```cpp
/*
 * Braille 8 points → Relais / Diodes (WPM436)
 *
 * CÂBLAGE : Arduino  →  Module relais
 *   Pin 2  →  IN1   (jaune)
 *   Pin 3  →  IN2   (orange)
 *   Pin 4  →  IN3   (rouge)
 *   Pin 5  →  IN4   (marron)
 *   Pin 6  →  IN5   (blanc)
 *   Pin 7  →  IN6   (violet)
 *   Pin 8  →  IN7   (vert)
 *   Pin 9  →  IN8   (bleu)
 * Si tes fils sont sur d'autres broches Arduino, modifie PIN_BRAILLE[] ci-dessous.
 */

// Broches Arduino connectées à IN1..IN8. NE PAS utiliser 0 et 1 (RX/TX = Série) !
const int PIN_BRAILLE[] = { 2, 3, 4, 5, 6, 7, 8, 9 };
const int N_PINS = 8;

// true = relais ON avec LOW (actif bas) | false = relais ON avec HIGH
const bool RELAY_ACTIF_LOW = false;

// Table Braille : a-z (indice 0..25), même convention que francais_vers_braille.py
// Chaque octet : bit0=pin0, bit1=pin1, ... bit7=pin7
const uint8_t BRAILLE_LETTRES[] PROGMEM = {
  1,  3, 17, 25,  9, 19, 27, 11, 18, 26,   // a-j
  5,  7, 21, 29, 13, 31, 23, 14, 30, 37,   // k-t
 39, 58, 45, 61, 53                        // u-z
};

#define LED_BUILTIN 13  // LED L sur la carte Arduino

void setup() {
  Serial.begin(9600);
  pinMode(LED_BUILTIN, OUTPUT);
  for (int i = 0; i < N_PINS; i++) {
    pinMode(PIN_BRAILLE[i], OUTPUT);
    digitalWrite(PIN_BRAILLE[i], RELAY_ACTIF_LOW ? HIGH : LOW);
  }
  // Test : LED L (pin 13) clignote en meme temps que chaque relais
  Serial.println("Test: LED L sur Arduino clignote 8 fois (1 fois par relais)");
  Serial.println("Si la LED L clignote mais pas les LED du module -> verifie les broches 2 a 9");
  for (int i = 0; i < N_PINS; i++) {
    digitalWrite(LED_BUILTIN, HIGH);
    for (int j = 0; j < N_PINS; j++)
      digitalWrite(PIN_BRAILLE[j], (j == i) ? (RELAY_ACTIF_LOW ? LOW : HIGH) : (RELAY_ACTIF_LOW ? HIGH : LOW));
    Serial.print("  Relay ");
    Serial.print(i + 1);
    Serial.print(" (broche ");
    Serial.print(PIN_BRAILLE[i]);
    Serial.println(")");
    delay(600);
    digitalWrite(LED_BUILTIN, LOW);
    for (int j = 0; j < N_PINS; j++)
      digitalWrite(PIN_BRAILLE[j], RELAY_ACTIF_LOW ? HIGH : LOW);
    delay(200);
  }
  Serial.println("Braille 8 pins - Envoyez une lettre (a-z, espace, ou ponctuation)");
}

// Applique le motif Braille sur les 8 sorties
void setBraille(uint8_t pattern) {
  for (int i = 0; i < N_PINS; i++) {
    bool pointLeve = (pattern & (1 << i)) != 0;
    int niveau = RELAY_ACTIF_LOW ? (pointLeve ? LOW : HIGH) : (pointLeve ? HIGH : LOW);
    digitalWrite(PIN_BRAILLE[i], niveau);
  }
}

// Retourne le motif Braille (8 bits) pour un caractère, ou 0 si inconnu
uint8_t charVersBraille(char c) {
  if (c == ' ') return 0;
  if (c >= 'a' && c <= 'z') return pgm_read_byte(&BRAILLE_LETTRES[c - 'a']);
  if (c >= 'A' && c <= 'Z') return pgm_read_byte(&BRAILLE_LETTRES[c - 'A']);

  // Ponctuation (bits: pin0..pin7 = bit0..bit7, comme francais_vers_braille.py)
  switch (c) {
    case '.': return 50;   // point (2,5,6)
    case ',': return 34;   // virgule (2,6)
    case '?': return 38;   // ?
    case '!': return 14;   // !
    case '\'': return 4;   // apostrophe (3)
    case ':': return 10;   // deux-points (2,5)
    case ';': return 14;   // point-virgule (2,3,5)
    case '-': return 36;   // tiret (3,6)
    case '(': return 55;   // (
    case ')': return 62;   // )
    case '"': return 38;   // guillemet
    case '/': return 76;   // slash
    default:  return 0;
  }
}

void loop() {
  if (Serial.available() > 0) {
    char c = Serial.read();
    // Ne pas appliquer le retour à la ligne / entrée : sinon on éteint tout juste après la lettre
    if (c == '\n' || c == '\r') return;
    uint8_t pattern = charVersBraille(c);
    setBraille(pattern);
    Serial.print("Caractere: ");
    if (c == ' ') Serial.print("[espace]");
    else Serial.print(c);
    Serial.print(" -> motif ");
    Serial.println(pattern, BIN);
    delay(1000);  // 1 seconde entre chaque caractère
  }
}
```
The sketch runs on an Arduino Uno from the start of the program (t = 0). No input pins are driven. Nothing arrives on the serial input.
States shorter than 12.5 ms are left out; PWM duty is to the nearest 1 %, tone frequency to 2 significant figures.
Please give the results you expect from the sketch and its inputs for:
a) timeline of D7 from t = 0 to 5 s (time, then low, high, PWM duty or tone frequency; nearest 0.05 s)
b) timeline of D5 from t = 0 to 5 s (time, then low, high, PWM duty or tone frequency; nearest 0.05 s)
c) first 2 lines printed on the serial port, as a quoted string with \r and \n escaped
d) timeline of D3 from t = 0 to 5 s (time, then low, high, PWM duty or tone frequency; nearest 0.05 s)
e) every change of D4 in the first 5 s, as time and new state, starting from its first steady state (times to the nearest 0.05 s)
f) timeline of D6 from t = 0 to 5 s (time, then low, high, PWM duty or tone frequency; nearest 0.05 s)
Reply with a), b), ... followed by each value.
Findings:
a) 0 s low; 4.1 s high; 4.7 s low
b) 0 s low; 2.5 s high; 3.1 s low
c) "Test: LED L sur Arduino clignote 8 fois (1 fois par relais)\r\nSi la LED L clignote mais pas les LED du module -> verifie les broches 2 a 9\r\n"
d) 0 s low; 0.9 s high; 1.5 s low
e) 0 s low; 1.7 s high; 2.3 s low
f) 0 s low; 3.3 s high; 3.9 s low
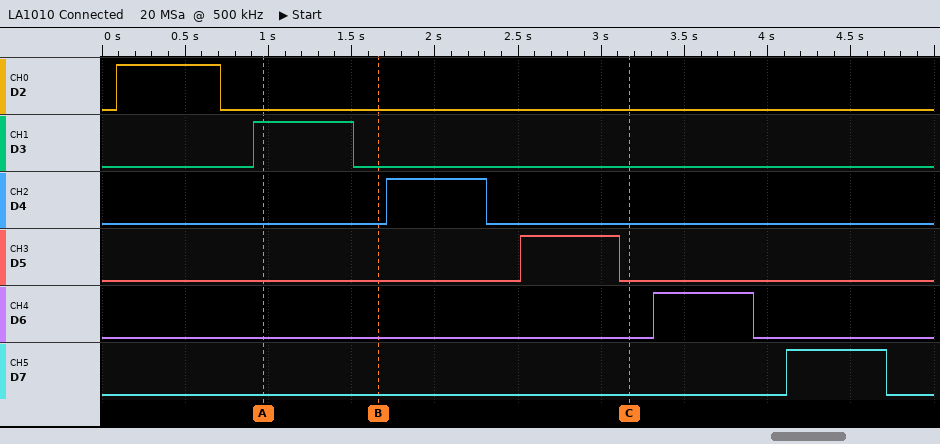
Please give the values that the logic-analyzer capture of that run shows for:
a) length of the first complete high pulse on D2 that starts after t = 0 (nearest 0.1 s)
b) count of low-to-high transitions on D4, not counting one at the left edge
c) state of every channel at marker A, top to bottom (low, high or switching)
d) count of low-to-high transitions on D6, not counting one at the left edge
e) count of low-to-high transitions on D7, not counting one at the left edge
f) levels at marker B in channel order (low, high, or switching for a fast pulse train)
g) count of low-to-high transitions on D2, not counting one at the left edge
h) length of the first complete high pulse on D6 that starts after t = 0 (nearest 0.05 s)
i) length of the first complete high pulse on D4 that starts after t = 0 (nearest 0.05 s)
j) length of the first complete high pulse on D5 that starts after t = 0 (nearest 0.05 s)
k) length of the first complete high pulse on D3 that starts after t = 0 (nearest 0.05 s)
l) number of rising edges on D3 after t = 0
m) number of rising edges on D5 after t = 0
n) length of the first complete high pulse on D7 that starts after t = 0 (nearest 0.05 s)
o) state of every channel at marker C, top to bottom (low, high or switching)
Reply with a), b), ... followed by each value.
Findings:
a) 0.6 s
b) 1
c) D2 low, D3 high, D4 low, D5 low, D6 low, D7 low
d) 1
e) 1
f) D2 low, D3 low, D4 low, D5 low, D6 low, D7 low
g) 1
h) 0.60 s
i) 0.60 s
j) 0.60 s
k) 0.60 s
l) 1
m) 1
n) 0.60 s
o) D2 low, D3 low, D4 low, D5 low, D6 low, D7 low
